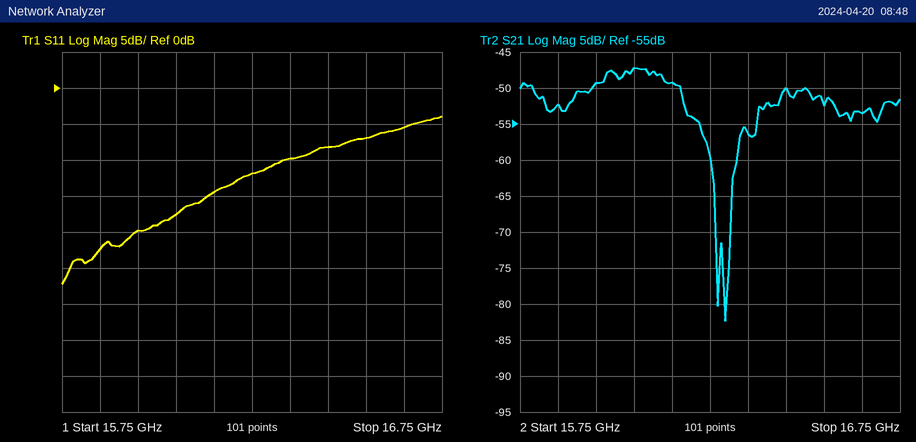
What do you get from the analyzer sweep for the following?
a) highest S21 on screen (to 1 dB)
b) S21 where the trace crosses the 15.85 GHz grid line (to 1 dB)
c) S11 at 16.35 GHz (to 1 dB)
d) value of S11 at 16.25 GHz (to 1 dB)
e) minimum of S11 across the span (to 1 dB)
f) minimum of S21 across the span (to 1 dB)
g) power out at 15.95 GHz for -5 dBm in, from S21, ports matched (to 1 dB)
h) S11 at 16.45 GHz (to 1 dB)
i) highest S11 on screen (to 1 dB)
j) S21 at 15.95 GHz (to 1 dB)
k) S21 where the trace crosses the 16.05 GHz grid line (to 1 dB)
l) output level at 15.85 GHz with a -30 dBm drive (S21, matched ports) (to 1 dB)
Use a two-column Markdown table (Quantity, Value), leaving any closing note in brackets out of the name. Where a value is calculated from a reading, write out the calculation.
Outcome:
| Quantity | Value |
|---|---|
| highest S21 on screen | -47 dB |
| S21 where the trace crosses the 15.85 GHz grid line | -52 dB |
| S11 at 16.35 GHz | -10 dB |
| value of S11 at 16.25 GHz | -12 dB |
| minimum of S11 across the span | -27 dB |
| minimum of S21 across the span | -82 dB |
| power out at 15.95 GHz for -5 dBm in, from S21, ports matched | -5 dBm + (-49 dB) = -54 dBm |
| S11 at 16.45 GHz | -8 dB |
| highest S11 on screen | -4 dB |
| S21 at 15.95 GHz | -49 dB |
| S21 where the trace crosses the 16.05 GHz grid line | -47 dB |
| output level at 15.85 GHz with a -30 dBm drive (S21, matched ports) | -30 dBm + (-52 dB) = -82 dBm |
